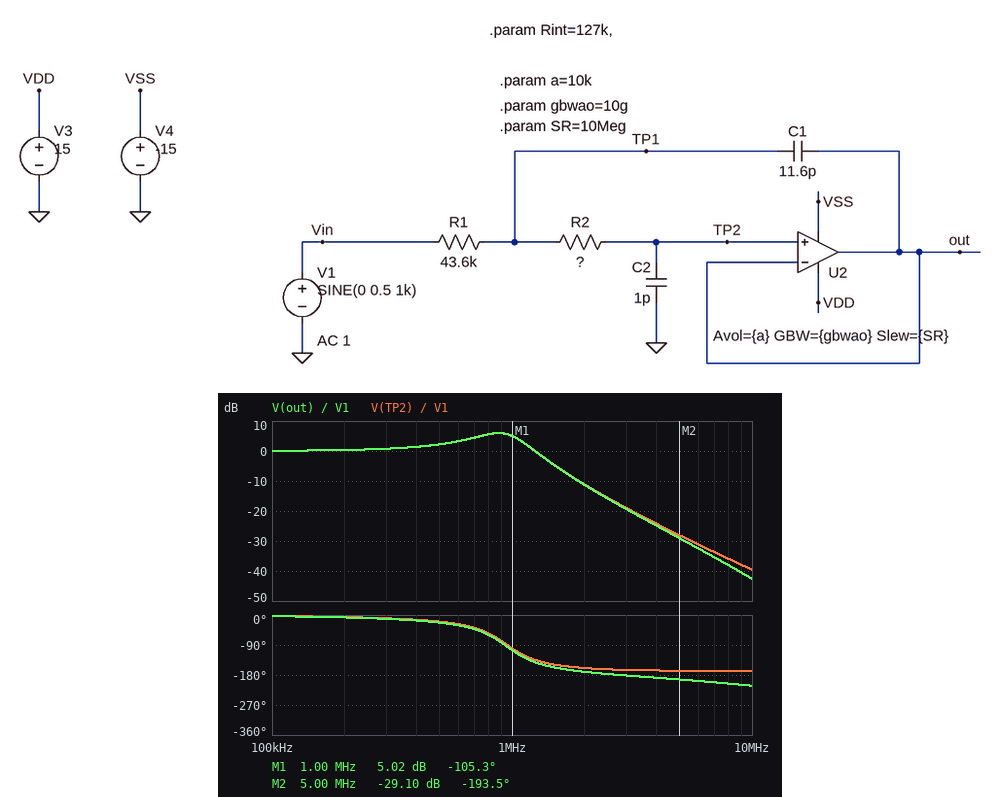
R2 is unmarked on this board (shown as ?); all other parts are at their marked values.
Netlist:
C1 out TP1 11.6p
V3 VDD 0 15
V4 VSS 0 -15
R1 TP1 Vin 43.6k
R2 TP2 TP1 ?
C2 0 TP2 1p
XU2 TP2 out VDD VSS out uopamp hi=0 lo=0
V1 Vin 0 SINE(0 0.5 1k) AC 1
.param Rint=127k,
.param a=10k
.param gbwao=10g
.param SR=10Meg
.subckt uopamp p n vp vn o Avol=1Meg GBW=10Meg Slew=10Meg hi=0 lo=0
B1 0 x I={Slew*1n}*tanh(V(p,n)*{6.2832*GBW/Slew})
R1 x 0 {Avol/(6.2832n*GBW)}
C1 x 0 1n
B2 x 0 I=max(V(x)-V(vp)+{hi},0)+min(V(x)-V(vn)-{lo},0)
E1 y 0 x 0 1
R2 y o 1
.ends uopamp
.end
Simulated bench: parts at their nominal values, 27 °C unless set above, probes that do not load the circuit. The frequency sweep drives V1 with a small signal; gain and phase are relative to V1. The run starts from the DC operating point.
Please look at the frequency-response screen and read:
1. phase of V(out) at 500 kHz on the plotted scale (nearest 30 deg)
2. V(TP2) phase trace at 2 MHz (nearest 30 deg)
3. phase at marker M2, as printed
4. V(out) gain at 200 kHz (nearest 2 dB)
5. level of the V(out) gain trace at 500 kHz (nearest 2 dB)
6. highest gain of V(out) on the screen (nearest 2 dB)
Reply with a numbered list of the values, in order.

1. -30 deg
2. -150 deg
3. -193.5 deg
4. 0 dB
5. 2 dB
6. 6 dB
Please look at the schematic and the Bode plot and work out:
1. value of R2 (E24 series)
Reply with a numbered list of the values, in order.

1. 39 kΩ
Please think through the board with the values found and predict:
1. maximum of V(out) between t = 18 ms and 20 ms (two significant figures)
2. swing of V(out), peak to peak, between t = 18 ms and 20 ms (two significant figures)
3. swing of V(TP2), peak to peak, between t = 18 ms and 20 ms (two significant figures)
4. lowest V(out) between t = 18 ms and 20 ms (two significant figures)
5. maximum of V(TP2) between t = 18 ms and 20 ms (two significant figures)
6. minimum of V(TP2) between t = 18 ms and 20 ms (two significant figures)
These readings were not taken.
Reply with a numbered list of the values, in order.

1. 500 mV
2. 1.0 V
3. 1.0 V
4. -500 mV
5. 500 mV
6. -500 mV
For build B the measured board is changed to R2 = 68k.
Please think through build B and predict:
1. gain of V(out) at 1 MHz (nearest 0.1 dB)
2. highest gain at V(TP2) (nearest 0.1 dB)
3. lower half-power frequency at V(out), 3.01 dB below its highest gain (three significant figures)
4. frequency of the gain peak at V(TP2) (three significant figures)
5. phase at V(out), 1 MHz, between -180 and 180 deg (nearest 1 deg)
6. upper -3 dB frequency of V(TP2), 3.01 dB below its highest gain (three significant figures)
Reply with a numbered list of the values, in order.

1. 0 dB
2. 5.5 dB
3. 430 kHz
4. 708 kHz
5. -138 deg
6. 904 kHz
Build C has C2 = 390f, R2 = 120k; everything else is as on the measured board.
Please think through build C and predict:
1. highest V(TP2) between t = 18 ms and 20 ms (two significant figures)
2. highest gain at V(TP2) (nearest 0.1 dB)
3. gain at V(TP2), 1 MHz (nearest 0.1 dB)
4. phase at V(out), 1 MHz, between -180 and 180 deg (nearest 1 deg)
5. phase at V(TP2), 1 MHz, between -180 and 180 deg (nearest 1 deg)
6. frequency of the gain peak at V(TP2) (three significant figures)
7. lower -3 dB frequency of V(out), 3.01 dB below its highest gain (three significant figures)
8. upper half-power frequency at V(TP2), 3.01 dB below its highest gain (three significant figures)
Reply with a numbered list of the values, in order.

1. 500 mV
2. 8.6 dB
3. 6.0 dB
4. -126 deg
5. -120 deg
6. 858 kHz
7. 663 kHz
8. 1.02 MHz
